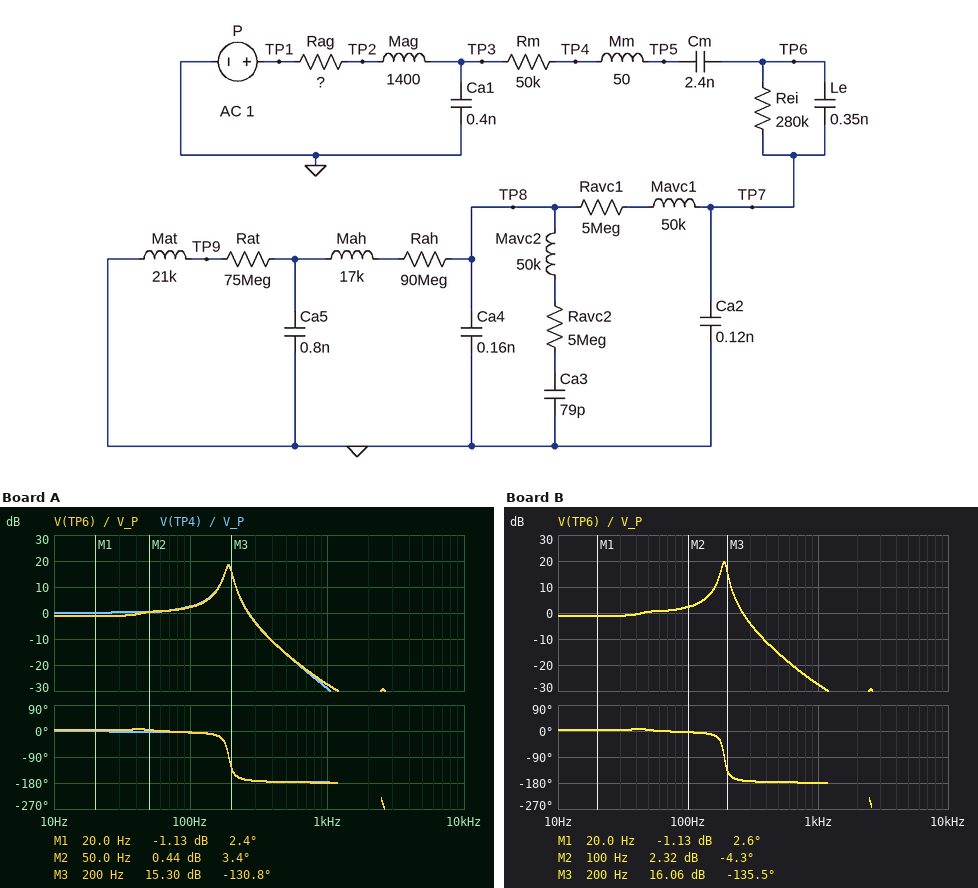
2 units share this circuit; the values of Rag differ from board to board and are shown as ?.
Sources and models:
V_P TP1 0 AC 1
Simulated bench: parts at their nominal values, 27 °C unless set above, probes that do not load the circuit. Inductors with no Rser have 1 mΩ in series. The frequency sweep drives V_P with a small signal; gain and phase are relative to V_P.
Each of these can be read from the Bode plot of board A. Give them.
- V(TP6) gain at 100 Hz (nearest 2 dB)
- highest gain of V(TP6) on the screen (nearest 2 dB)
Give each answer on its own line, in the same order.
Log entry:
2 dB
18 dB
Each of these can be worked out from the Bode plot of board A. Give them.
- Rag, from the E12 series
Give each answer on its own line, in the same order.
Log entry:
180 kΩ
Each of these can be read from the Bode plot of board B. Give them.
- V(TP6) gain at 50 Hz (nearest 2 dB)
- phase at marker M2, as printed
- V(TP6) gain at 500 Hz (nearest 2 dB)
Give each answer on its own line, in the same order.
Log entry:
0 dB
-4.3 deg
-16 dB
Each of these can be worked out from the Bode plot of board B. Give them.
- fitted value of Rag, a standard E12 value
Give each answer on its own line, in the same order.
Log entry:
150 kΩ
